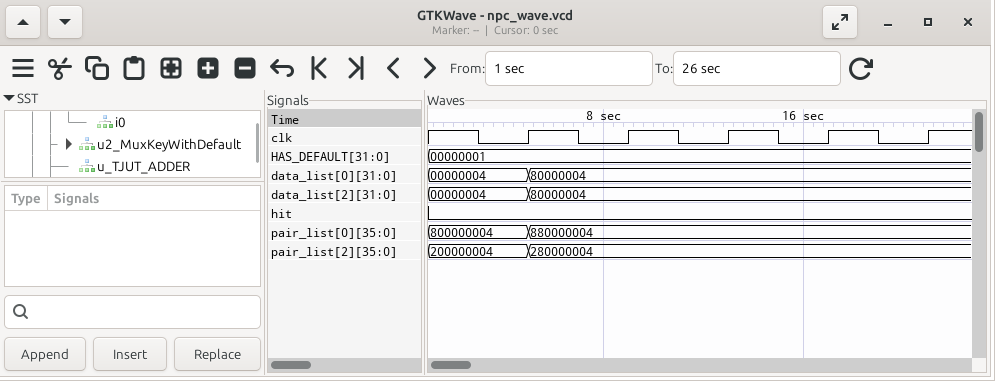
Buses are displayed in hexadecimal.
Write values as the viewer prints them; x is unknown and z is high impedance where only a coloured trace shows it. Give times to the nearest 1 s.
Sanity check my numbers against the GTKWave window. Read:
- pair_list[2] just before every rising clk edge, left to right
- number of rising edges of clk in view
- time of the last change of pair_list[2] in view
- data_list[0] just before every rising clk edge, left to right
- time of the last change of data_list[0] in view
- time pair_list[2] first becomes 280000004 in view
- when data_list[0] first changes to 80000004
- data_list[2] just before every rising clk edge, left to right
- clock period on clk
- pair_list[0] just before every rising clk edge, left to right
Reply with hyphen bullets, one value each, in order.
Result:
- 200000004, 280000004, 280000004, 280000004, 280000004
- 5
- 5 s
- 00000004, 80000004, 80000004, 80000004, 80000004
- 5 s
- 5 s
- 5 s
- 00000004, 80000004, 80000004, 80000004, 80000004
- 4 s
- 800000004, 880000004, 880000004, 880000004, 880000004
